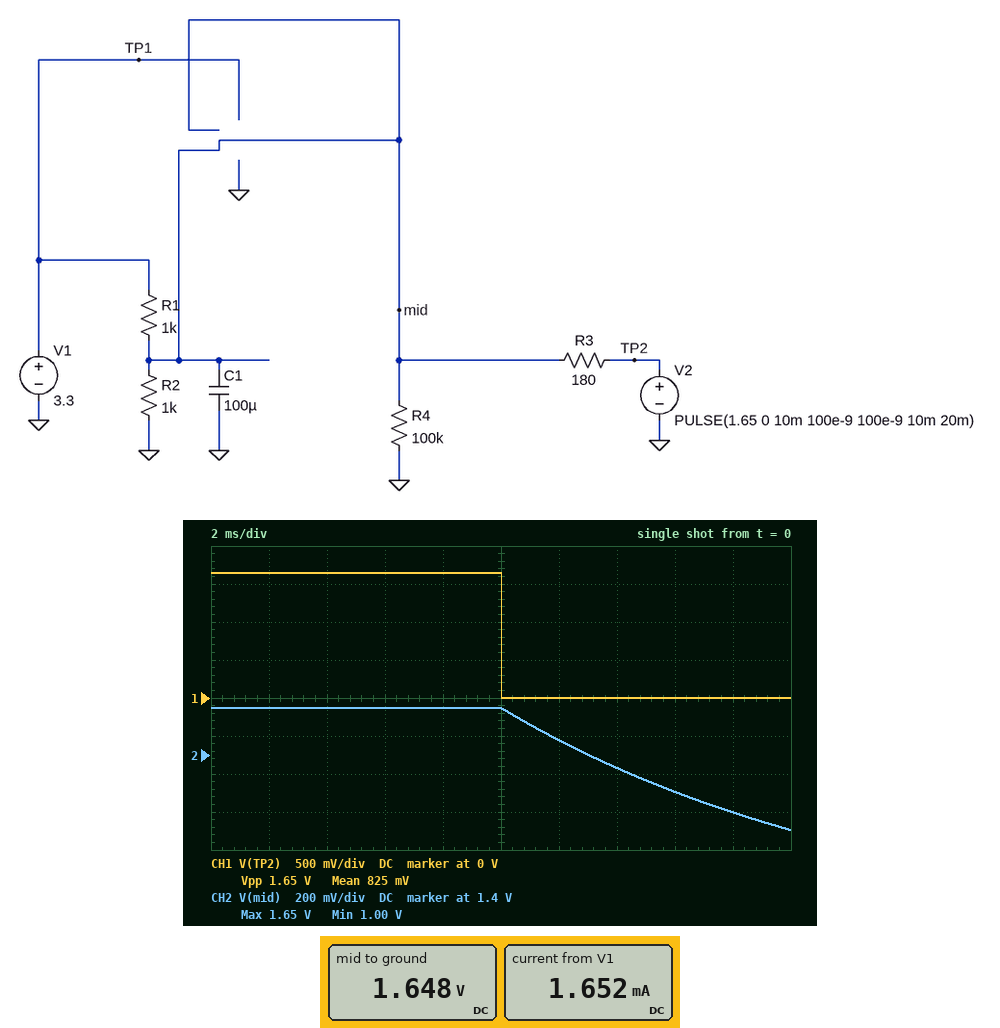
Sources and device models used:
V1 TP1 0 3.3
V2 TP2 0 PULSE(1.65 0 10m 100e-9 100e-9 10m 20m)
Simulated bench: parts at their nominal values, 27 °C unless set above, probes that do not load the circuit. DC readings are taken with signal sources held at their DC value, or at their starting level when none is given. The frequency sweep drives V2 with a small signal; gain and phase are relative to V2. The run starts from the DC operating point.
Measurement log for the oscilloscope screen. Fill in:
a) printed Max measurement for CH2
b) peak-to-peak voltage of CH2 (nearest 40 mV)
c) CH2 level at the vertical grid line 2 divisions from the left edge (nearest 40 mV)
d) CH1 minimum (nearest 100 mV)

1.65 V
640 mV
1.64 V
0 V
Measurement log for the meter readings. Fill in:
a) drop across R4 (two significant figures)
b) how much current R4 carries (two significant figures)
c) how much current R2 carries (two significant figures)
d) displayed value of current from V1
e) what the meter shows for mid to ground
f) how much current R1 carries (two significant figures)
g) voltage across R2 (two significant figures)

1.6 V
16 µA
1.6 mA
1.652 mA
1.648 V
1.7 mA
1.6 V
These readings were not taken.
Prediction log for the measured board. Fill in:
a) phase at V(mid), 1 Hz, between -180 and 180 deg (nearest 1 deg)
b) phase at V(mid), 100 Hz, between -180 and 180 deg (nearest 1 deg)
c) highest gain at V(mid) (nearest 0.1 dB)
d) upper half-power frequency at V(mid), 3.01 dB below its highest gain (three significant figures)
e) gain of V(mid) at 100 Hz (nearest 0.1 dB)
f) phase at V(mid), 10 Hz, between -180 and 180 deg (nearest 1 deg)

-5 deg
-83 deg
-2.7 dB
12.0 Hz
-21.1 dB
-40 deg
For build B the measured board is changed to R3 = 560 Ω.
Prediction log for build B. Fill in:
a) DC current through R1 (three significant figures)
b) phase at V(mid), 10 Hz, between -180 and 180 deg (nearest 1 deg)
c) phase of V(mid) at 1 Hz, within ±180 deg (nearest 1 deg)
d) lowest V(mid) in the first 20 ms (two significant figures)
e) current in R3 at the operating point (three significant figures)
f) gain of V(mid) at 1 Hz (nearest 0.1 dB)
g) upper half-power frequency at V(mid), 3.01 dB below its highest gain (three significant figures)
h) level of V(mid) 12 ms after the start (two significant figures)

1.65 mA
-59 deg
-9 deg
1.4 V
7.76 µA
-6.7 dB
6.04 Hz
1.6 V
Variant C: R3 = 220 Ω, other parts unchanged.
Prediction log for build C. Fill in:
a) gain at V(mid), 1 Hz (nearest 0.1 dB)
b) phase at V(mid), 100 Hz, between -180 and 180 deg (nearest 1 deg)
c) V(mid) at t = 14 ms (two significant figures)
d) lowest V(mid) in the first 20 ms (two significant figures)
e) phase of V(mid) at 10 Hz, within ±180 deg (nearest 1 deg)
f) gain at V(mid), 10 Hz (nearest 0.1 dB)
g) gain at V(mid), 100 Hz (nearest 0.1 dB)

-3.2 dB
-84 deg
1.4 V
1.1 V
-44 deg
-6.0 dB
-22.9 dB
